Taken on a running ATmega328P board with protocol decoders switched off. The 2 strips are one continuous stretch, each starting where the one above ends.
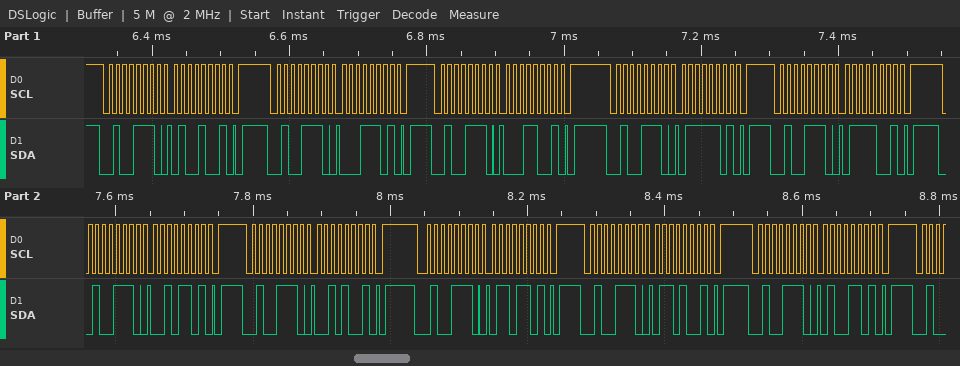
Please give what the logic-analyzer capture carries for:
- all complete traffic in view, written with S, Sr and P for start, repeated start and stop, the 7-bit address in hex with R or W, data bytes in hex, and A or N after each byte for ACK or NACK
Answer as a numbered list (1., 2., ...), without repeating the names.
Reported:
1. S 27W A 49 A P S 27W A 1D A P S 27W A 19 A P S 27W A 7D A P S 27W A 79 A P S 27W A 2D A P S 27W A 29 A P S 27W A 6D A P S 27W A 69 A P S 27W A 4D A P
